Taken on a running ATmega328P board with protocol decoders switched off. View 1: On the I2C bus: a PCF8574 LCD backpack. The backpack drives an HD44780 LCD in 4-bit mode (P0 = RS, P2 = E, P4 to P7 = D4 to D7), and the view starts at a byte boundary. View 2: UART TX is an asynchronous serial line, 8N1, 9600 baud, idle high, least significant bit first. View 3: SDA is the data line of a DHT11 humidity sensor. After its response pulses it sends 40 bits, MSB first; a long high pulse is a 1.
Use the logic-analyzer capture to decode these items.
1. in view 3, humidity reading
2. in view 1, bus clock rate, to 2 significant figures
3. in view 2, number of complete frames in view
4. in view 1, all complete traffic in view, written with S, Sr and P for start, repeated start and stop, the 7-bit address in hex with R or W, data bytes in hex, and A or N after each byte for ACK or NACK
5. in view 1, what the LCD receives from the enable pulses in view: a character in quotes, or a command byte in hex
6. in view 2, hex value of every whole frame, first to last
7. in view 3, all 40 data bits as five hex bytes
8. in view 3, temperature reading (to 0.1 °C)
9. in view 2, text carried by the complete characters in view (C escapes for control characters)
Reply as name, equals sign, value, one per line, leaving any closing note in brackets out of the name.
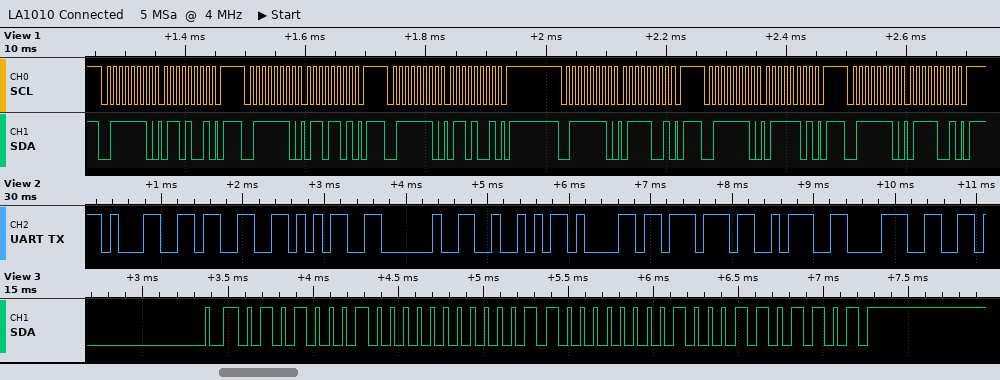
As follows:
in view 3, humidity reading = 81 %
in view 1, bus clock rate, to 2 significant figures = 100 kHz
in view 2, number of complete frames in view = 9
in view 1, all complete traffic in view, written with S, Sr and P for start, repeated start and stop, the 7-bit address in hex with R or W, data bytes in hex, and A or N after each byte for ACK or NACK = S 3FW A 69 A P S 3FW A 6D A P S 3FW A 69 A P S 3FW A 79 A P S 3FW A 7D A P S 3FW A 79 A P
in view 1, what the LCD receives from the enable pulses in view: a character in quotes, or a command byte in hex = 'g'
in view 2, hex value of every whole frame, first to last = 31 33 35 20 52 61 77 3A 38
in view 3, all 40 data bits as five hex bytes = 51 00 18 04 6D
in view 3, temperature reading = 24.4 °C
in view 2, text carried by the complete characters in view = "135 Raw:8"
